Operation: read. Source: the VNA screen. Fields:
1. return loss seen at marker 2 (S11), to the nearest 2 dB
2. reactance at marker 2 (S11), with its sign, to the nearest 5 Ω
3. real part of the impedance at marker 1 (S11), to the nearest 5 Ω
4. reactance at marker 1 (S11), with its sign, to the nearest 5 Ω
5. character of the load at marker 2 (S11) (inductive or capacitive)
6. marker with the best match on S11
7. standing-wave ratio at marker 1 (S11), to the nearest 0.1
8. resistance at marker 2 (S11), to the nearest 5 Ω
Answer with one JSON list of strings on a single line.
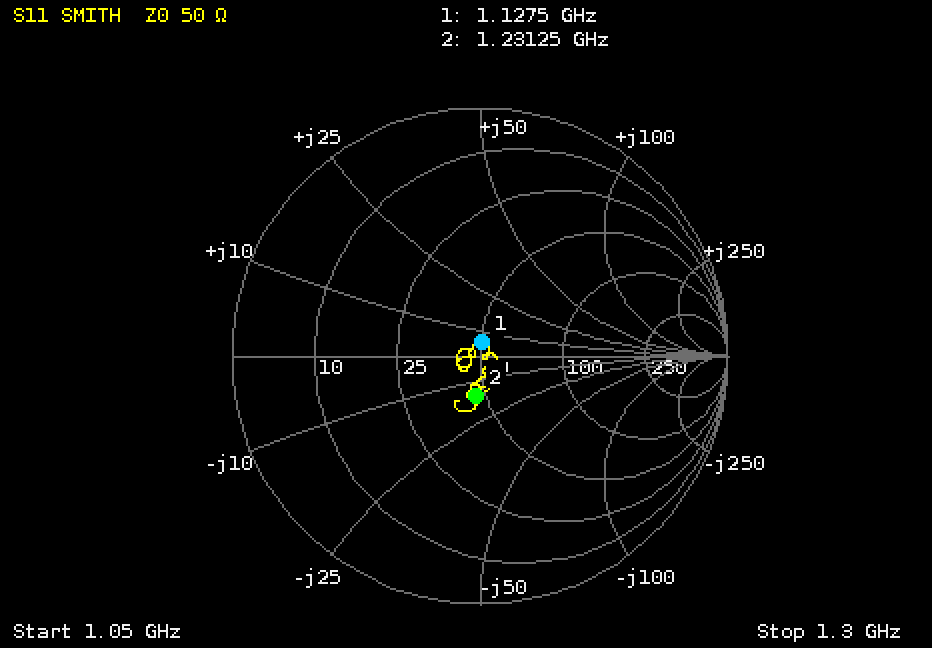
["16 dB", "-15 Ω", "50 Ω", "+5 Ω", "capacitive", "marker 1", "1.1", "45 Ω"]
